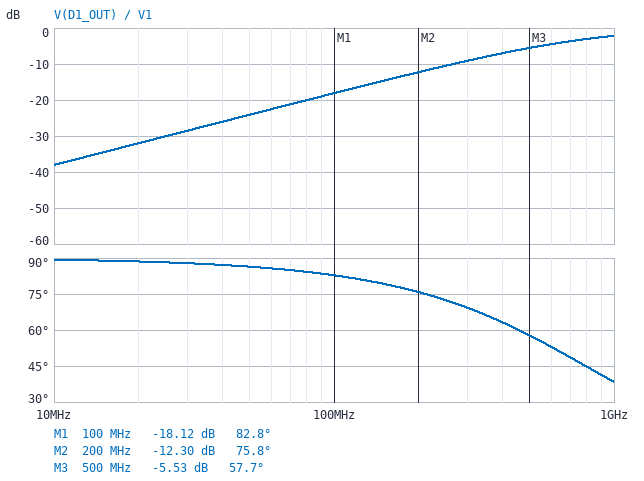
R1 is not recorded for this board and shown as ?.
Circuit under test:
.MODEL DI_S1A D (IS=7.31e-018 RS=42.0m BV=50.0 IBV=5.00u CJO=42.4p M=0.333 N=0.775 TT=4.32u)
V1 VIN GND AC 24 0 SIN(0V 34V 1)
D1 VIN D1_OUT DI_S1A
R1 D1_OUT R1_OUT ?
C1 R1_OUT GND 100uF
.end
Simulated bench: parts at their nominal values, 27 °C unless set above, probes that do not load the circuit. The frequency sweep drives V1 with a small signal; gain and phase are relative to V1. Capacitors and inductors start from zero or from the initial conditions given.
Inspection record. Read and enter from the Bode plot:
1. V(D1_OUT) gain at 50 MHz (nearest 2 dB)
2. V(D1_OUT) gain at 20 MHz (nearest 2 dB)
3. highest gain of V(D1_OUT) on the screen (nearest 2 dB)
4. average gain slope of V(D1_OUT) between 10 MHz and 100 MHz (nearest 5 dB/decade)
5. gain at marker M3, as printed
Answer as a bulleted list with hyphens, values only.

- -24 dB
- -32 dB
- -2 dB
- 20 dB/decade
- -5.53 dB
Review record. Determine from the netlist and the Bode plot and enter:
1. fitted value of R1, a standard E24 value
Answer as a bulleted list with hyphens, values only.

- 4.7 Ω
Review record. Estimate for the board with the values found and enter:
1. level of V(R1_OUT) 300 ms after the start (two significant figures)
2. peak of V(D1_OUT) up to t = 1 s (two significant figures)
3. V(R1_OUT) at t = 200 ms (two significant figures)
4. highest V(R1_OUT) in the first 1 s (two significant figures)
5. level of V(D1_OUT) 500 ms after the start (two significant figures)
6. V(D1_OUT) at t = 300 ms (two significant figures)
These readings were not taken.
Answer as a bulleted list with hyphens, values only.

- 33 V
- 33 V
- 32 V
- 33 V
- 33 V
- 33 V
